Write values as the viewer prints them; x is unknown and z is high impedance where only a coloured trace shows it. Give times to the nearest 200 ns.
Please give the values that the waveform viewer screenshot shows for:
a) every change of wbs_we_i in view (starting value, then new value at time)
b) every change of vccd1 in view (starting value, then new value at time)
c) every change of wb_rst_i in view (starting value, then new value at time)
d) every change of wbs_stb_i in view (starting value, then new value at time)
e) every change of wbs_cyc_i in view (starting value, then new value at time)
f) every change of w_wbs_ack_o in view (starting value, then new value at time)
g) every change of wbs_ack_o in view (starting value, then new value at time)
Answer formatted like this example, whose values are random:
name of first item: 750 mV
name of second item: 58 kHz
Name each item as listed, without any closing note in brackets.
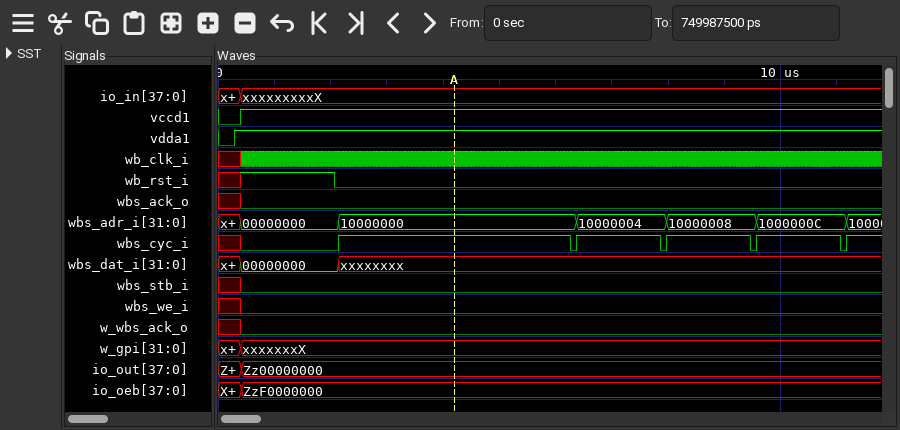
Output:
every change of wbs_we_i in view: x, 0 at 400 ns
every change of vccd1 in view: 0, 1 at 400 ns
every change of wb_rst_i in view: x, 1 at 400 ns, 0 at 2000 ns
every change of wbs_stb_i in view: x, 0 at 400 ns
every change of wbs_cyc_i in view: x, 0 at 400 ns, 1 at 2200 ns, 0 at 6200 ns, 1 at 6400 ns, 0 at 7800 ns, 1 at 8000 ns, 0 at 9400 ns, 1 at 9600 ns, 0 at 11000 ns, 1 at 11200 ns
every change of w_wbs_ack_o in view: x, 0 at 400 ns
every change of wbs_ack_o in view: x, 0 at 400 ns
